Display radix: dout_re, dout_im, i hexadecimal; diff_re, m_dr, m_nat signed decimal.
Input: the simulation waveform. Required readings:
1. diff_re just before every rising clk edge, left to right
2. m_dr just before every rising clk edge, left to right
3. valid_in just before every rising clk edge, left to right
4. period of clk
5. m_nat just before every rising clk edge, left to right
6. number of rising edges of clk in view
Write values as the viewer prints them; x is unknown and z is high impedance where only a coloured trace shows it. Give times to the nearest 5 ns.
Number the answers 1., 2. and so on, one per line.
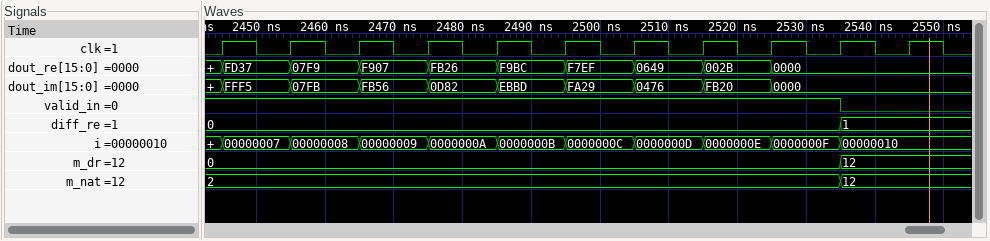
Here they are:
1. 0, 0, 0, 0, 0, 0, 0, 0, 0, 0, 1
2. 0, 0, 0, 0, 0, 0, 0, 0, 0, 0, 12
3. 1 1 1 1 1 1 1 1 1 1 0
4. 10 ns
5. 2, 2, 2, 2, 2, 2, 2, 2, 2, 2, 12
6. 11
